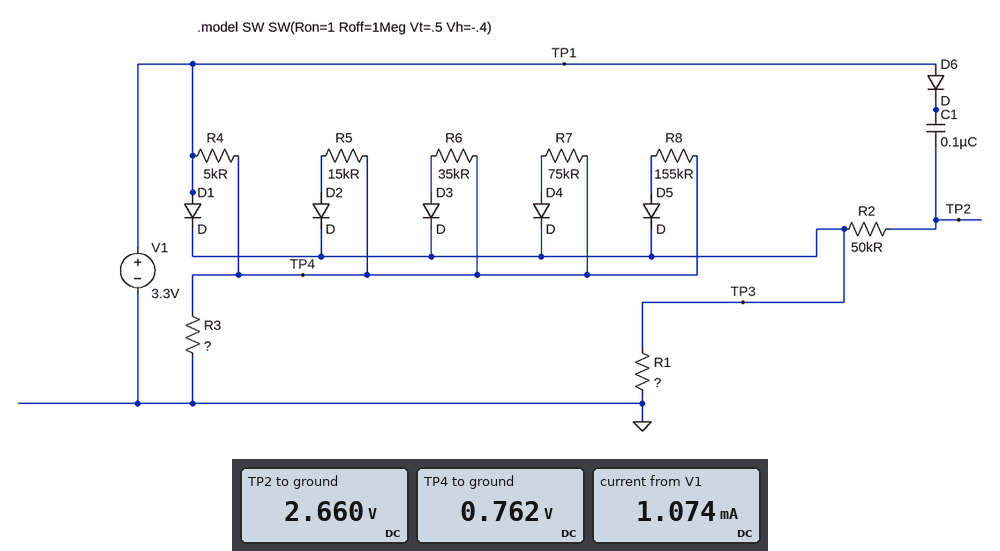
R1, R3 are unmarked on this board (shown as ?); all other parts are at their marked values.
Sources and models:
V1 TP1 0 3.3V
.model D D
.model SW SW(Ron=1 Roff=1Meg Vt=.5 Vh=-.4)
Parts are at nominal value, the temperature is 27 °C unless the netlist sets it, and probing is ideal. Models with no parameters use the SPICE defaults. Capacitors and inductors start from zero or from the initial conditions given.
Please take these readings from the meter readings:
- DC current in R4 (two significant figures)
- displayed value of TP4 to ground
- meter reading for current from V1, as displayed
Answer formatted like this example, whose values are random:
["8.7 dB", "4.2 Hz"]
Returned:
["510 µA", "0.762 V", "1.074 mA"]
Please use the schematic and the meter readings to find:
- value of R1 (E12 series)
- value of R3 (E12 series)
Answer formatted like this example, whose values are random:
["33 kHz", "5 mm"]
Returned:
["4.7 kΩ", "1.5 kΩ"]
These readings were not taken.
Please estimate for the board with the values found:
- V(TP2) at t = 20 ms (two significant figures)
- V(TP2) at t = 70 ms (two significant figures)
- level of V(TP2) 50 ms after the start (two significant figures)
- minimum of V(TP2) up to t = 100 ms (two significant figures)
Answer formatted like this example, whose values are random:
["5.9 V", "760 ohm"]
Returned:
["2.7 V", "2.7 V", "2.7 V", "2.7 V"]
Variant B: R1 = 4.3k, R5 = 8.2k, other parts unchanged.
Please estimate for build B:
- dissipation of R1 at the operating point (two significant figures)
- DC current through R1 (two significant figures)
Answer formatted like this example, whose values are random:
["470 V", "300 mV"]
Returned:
["1.6 mW", "620 µA"]
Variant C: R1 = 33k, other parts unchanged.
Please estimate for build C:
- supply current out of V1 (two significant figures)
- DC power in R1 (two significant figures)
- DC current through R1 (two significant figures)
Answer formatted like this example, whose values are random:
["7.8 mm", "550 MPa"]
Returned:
["590 µA", "220 µW", "82 µA"]
